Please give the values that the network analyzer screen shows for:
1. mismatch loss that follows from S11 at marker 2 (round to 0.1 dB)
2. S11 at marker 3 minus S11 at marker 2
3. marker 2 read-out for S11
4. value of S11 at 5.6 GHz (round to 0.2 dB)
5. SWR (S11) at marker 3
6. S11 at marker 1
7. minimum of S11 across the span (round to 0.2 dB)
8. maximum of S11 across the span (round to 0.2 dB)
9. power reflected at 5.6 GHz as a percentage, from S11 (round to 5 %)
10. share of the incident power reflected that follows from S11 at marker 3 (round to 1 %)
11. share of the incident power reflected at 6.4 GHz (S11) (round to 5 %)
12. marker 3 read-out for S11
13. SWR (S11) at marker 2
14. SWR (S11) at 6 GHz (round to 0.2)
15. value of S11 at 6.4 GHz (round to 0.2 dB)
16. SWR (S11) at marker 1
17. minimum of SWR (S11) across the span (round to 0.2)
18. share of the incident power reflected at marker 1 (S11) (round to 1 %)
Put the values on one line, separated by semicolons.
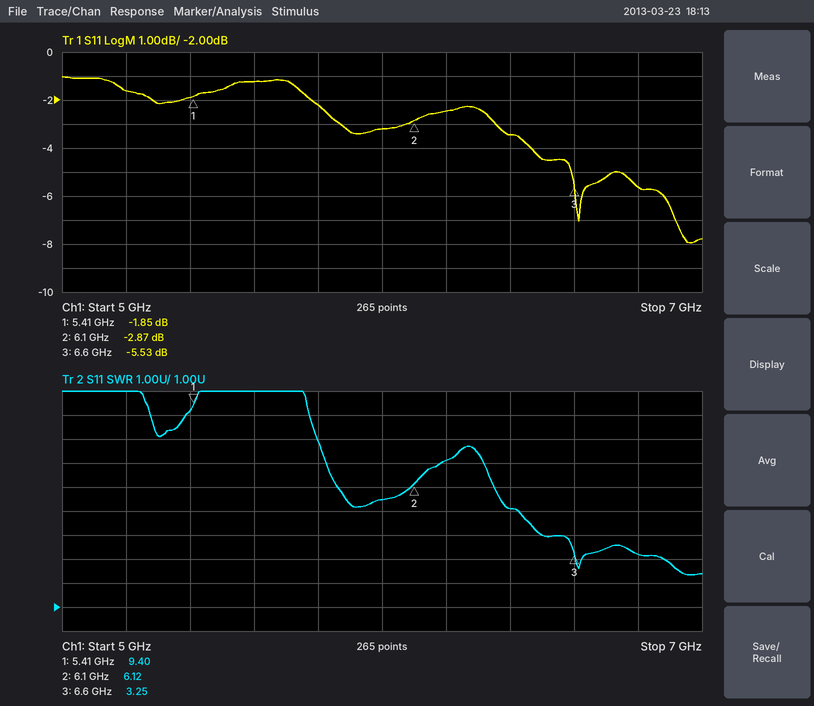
3.2 dB; -2.66 dB; -2.87 dB; -1.2 dB; 3.25; -1.85 dB; -8.0 dB; -1.0 dB; 75 %; 28 %; 45 %; -5.53 dB; 6.12; 5.4; -3.4 dB; 9.40; 2.4; 65 %
